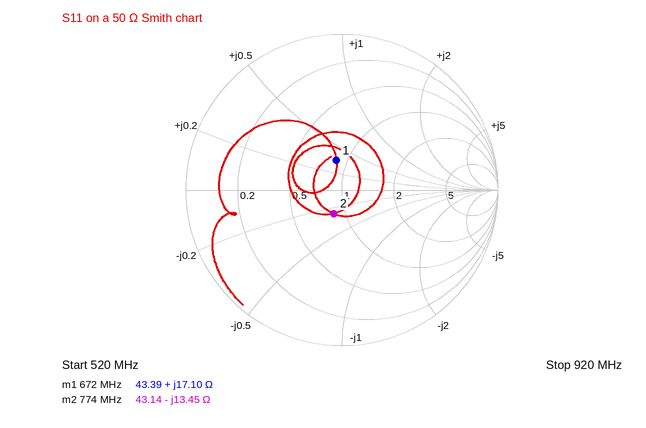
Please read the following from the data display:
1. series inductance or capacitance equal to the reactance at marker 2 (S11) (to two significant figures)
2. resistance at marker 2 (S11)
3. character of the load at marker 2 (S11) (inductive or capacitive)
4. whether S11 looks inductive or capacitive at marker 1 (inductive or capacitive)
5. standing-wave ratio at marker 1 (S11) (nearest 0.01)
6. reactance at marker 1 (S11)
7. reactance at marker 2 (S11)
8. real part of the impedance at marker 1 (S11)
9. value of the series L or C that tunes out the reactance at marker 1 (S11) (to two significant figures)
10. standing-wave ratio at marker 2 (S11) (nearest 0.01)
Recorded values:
15 pF
43.14 Ω
capacitive
inductive
1.48
+17.10 Ω
-13.45 Ω
43.39 Ω
14 pF
1.38
